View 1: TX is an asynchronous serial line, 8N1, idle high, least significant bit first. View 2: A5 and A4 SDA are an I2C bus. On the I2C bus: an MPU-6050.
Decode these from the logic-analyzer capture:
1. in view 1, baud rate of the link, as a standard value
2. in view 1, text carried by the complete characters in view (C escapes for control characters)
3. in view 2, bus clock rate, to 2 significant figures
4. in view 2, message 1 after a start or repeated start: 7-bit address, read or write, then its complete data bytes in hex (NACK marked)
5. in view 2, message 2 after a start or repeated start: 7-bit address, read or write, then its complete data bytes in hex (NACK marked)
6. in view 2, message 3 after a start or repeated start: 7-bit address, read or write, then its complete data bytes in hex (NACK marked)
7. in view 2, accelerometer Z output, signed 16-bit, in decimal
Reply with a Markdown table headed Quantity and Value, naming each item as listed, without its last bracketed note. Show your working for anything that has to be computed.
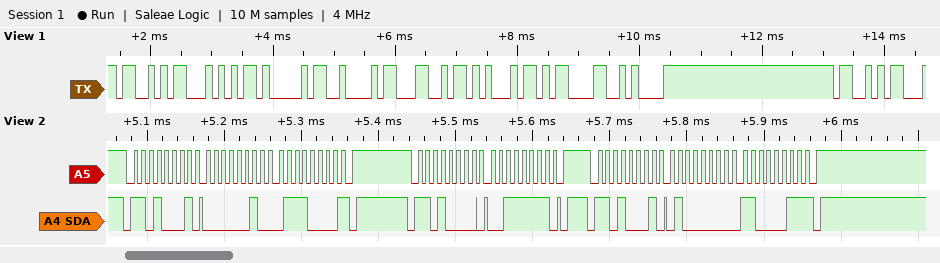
| Quantity | Value |
|---|---|
| in view 1, baud rate of the link, as a standard value | 9600 baud |
| in view 1, text carried by the complete characters in view | "STABLE\r\nS" |
| in view 2, bus clock rate, to 2 significant figures | 100 kHz |
| in view 2, message 1 after a start or repeated start: 7-bit address, read or write, then its complete data bytes in hex | 0x68 read: 02 70 NACK |
| in view 2, message 2 after a start or repeated start: 7-bit address, read or write, then its complete data bytes in hex | 0x68 write: 3F |
| in view 2, message 3 after a start or repeated start: 7-bit address, read or write, then its complete data bytes in hex | 0x68 read: 40 C3 NACK |
| in view 2, accelerometer Z output, signed 16-bit, in decimal | 0x40C3 = 16579 |
